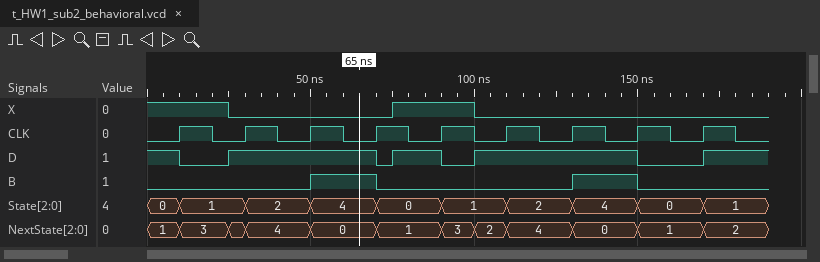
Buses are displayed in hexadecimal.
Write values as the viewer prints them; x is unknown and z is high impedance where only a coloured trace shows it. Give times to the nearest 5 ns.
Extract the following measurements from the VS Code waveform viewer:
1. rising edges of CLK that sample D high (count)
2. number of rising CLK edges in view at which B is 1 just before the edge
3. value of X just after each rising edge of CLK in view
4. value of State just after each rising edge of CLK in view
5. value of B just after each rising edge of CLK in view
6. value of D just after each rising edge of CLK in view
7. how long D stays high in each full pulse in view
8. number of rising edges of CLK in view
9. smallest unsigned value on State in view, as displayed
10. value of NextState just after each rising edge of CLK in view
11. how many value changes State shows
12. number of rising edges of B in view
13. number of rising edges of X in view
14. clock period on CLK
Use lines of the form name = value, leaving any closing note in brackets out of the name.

rising edges of CLK that sample D high = 8
number of rising CLK edges in view at which B is 1 just before the edge = 2
value of X just after each rising edge of CLK in view = 1 0 0 0 1 0 0 0 0
value of State just after each rising edge of CLK in view = 1, 2, 4, 0, 1, 2, 4, 0, 1
value of B just after each rising edge of CLK in view = 0 0 1 0 0 0 1 0 0
value of D just after each rising edge of CLK in view = 0 1 1 0 0 1 1 0 1
how long D stays high in each full pulse in view = 45 ns, 15 ns, 50 ns
number of rising edges of CLK in view = 9
smallest unsigned value on State in view, as displayed = 0
value of NextState just after each rising edge of CLK in view = 3, 4, 0, 1, 3, 4, 0, 1, 2
how many value changes State shows = 9
number of rising edges of B in view = 2
number of rising edges of X in view = 1
clock period on CLK = 20 ns
